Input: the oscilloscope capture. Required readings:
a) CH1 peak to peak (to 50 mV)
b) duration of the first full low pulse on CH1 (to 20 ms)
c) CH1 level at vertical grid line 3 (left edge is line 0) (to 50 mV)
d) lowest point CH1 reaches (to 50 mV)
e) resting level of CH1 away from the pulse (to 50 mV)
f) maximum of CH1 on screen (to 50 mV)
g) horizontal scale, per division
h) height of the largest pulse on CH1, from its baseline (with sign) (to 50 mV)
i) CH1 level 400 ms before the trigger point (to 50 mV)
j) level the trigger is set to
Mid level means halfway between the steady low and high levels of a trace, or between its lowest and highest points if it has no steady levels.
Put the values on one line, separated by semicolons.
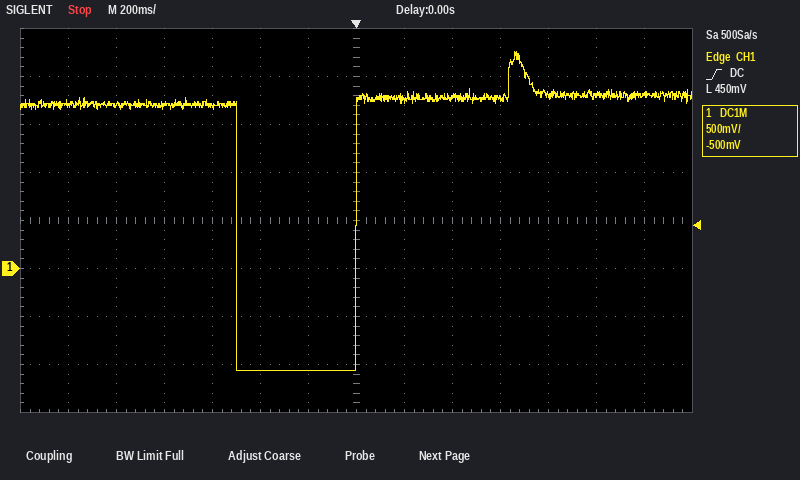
3.30 V; 500 ms; 1.70 V; -1.05 V; 1.75 V; 2.25 V; 200 ms; -2.80 V; -1.05 V; 450 mV
